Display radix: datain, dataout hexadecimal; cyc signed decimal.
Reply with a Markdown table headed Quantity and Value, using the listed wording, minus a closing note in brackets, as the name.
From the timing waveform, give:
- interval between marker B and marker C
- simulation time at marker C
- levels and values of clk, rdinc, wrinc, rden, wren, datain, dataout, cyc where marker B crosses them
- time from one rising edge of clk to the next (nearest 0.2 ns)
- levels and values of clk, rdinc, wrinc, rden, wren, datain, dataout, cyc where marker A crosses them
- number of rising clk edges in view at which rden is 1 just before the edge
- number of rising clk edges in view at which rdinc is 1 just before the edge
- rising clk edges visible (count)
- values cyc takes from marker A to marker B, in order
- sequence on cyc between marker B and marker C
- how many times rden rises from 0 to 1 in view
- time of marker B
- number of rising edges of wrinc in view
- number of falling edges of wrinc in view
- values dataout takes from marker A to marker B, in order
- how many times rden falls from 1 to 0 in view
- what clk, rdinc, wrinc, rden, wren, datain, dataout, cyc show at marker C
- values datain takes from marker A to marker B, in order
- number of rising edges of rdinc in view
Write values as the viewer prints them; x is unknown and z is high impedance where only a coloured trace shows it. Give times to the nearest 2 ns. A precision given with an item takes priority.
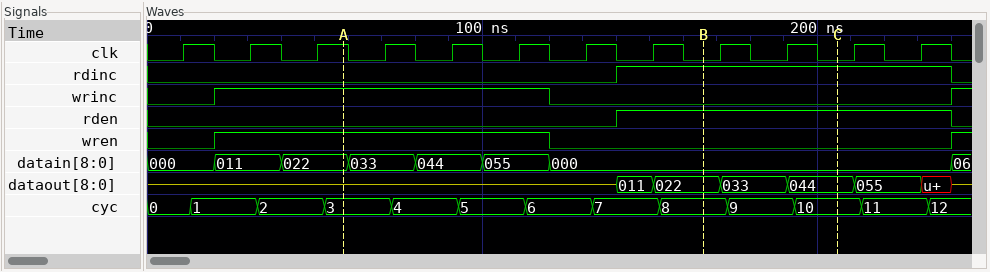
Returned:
| Quantity | Value |
|---|---|
| interval between marker B and marker C | 40 ns |
| simulation time at marker C | 206 ns |
| levels and values of clk, rdinc, wrinc, rden, wren, datain, dataout, cyc where marker B crosses them | clk=0, rdinc=1, wrinc=0, rden=1, wren=0, datain=000, dataout=022, cyc=8 |
| time from one rising edge of clk to the next | 20 ns |
| levels and values of clk, rdinc, wrinc, rden, wren, datain, dataout, cyc where marker A crosses them | clk=1, rdinc=0, wrinc=1, rden=0, wren=1, datain=022, dataout=z, cyc=3 |
| number of rising clk edges in view at which rden is 1 just before the edge | 5 |
| number of rising clk edges in view at which rdinc is 1 just before the edge | 5 |
| rising clk edges visible | 12 |
| values cyc takes from marker A to marker B, in order | 3, 4, 5, 6, 7, 8 |
| sequence on cyc between marker B and marker C | 8, 9, 10 |
| how many times rden rises from 0 to 1 in view | 1 |
| time of marker B | 166 ns |
| number of rising edges of wrinc in view | 2 |
| number of falling edges of wrinc in view | 1 |
| values dataout takes from marker A to marker B, in order | z, 011, 022 |
| how many times rden falls from 1 to 0 in view | 1 |
| what clk, rdinc, wrinc, rden, wren, datain, dataout, cyc show at marker C | clk=0, rdinc=1, wrinc=0, rden=1, wren=0, datain=000, dataout=044, cyc=10 |
| values datain takes from marker A to marker B, in order | 022, 033, 044, 055, 000 |
| number of rising edges of rdinc in view | 1 |
